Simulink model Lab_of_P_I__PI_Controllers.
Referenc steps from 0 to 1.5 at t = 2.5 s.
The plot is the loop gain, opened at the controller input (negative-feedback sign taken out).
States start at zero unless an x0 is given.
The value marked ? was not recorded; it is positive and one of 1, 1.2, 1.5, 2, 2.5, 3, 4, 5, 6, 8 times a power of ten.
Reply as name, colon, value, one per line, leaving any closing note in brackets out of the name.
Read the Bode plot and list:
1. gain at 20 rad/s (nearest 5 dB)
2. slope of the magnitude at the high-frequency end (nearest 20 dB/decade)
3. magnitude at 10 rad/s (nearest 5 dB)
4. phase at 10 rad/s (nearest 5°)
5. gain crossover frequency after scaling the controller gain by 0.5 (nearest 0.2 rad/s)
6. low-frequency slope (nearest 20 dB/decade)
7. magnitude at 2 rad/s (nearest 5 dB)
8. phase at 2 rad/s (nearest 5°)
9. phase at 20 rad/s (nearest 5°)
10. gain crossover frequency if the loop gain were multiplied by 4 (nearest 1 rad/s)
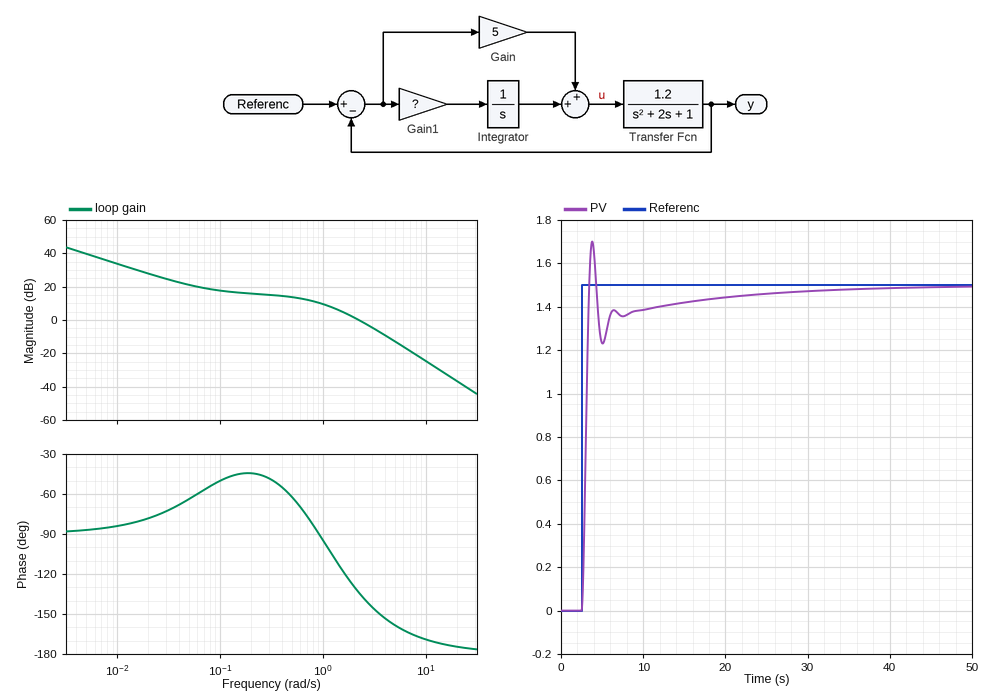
gain at 20 rad/s: -35 dB
slope of the magnitude at the high-frequency end: -40 dB/decade
magnitude at 10 rad/s: -25 dB
phase at 10 rad/s: -170°
gain crossover frequency after scaling the controller gain by 0.5: 1.4 rad/s
low-frequency slope: -20 dB/decade
magnitude at 2 rad/s: 0 dB
phase at 2 rad/s: -130°
phase at 20 rad/s: -175°
gain crossover frequency if the loop gain were multiplied by 4: 5 rad/s
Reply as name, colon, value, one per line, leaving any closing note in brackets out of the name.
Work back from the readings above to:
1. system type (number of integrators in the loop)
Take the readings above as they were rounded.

system type: 1
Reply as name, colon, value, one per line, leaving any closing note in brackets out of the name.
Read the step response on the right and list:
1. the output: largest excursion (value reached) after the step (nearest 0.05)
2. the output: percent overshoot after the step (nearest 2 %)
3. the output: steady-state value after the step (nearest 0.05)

the output: largest excursion (value reached) after the step: 1.70
the output: percent overshoot after the step: 14 %
the output: steady-state value after the step: 1.50
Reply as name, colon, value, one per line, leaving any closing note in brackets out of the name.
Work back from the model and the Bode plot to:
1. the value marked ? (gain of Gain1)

the value marked ?: 0.4
